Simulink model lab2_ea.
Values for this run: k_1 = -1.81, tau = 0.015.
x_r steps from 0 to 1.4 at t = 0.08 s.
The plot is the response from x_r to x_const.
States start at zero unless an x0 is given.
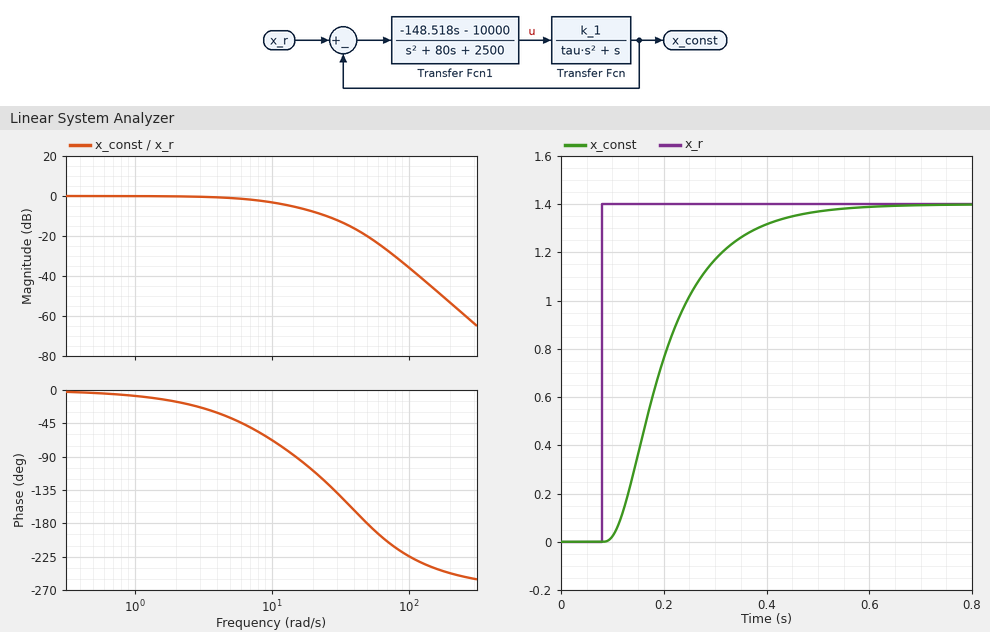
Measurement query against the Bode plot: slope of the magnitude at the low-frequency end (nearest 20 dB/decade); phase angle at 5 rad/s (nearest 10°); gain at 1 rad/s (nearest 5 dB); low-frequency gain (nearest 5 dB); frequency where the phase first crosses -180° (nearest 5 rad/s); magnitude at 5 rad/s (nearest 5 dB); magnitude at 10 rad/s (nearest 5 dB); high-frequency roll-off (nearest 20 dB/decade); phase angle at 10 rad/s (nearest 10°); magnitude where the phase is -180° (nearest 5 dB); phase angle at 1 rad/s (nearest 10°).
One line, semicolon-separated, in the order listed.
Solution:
0 dB/decade; -40°; 0 dB; 0 dB; 50 rad/s; 0 dB; -5 dB; -60 dB/decade; -70°; -20 dB; -10°
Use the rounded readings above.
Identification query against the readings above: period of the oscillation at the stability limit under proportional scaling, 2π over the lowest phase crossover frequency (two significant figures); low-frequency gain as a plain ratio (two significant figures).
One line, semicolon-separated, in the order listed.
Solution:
0.13 s; 1.0
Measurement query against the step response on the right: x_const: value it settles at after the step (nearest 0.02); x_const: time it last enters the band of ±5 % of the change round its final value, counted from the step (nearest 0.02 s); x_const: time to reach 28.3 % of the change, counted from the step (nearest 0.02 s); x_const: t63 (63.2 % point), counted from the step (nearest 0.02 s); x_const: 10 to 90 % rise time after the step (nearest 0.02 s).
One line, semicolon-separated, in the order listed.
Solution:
1.40; 0.34 s; 0.08 s; 0.14 s; 0.22 s
